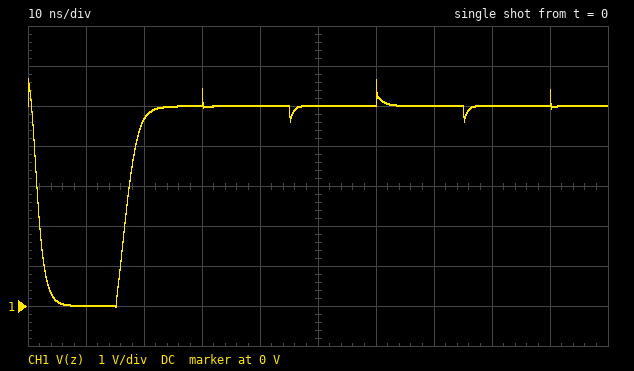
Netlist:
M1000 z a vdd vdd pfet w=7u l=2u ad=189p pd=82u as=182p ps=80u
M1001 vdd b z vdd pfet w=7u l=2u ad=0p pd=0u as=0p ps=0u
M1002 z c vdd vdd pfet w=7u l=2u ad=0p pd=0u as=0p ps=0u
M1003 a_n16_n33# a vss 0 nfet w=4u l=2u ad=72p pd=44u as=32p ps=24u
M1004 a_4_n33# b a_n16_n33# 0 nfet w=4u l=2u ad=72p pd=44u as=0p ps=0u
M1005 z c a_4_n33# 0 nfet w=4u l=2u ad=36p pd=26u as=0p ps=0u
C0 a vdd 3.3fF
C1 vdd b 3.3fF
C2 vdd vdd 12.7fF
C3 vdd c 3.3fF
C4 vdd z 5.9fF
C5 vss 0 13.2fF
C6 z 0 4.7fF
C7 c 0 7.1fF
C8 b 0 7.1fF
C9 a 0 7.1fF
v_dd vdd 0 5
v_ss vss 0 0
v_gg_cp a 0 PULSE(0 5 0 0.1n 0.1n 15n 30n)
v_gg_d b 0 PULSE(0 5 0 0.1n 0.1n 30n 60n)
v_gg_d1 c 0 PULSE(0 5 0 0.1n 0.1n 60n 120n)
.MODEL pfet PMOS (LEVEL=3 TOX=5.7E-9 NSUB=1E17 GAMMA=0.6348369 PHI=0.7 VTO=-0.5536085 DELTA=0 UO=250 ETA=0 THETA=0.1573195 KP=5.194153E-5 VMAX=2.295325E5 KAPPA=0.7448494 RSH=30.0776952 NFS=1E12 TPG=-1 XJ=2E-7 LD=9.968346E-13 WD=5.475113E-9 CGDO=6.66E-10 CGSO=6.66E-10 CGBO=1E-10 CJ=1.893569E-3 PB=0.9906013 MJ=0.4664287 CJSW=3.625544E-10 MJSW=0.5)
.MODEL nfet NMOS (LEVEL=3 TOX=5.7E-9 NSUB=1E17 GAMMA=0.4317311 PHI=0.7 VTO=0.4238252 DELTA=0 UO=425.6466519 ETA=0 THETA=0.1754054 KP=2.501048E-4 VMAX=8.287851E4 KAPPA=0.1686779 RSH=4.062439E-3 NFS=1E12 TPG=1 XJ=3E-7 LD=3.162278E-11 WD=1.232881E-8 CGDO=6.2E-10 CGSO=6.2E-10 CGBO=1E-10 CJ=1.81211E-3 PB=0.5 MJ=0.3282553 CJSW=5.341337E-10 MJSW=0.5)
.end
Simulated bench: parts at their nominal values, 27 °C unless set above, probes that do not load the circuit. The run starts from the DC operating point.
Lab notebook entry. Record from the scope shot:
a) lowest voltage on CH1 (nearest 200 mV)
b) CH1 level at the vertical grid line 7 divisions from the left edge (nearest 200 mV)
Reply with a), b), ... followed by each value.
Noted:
a) 0 V
b) 5.0 V
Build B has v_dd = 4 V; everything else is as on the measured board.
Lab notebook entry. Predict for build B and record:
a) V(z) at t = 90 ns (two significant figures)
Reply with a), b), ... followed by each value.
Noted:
a) 4.0 V
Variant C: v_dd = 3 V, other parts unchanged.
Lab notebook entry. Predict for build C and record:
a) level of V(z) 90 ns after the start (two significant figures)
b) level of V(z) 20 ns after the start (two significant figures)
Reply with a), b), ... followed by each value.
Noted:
a) 3.0 V
b) 2.0 V
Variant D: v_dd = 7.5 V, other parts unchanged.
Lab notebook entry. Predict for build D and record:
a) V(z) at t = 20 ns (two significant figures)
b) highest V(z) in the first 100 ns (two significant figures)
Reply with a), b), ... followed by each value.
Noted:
a) 7.5 V
b) 8.2 V
